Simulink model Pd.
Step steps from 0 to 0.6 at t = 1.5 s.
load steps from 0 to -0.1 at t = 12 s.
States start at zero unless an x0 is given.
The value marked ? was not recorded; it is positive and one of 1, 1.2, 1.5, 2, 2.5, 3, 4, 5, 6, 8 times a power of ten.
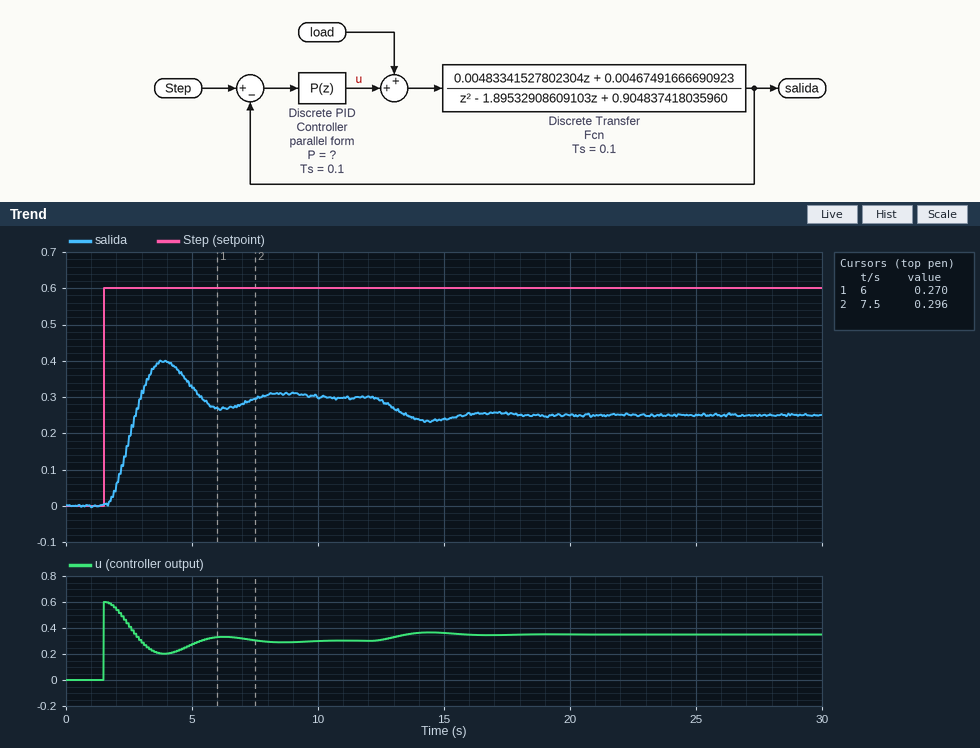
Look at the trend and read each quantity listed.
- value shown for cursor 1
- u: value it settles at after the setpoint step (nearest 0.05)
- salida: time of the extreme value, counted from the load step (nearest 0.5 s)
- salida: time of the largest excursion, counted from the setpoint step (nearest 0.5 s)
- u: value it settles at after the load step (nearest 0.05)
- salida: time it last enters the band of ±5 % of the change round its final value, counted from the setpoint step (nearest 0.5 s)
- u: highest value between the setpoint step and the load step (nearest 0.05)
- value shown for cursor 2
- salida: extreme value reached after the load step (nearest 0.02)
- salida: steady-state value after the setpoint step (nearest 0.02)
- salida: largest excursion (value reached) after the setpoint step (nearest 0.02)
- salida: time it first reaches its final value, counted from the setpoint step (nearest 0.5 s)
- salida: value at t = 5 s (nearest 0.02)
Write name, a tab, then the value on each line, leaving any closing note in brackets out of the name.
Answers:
value shown for cursor 1	0.270
u: value it settles at after the setpoint step	0.30
salida: time of the extreme value, counted from the load step	2.5 s
salida: time of the largest excursion, counted from the setpoint step	2.5 s
u: value it settles at after the load step	0.35
salida: time it last enters the band of ±5 % of the change round its final value, counted from the setpoint step	5.5 s
u: highest value between the setpoint step and the load step	0.60
value shown for cursor 2	0.296
salida: extreme value reached after the load step	0.24
salida: steady-state value after the setpoint step	0.30
salida: largest excursion (value reached) after the setpoint step	0.40
salida: time it first reaches its final value, counted from the setpoint step	1.5 s
salida: value at t = 5 s	0.32
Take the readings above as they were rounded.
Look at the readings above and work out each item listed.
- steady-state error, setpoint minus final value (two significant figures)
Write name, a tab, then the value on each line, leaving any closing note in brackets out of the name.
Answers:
steady-state error, setpoint minus final value	0.30
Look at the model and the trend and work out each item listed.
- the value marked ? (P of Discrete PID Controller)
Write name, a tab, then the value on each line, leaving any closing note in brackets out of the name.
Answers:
the value marked ?	1
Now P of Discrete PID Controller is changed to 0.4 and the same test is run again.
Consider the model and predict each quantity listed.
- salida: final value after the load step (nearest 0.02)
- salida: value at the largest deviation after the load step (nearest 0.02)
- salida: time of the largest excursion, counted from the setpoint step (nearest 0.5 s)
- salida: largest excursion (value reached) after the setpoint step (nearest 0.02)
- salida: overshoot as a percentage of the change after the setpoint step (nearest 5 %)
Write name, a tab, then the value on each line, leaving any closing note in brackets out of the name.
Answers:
salida: final value after the load step	0.10
salida: value at the largest deviation after the load step	0.08
salida: time of the largest excursion, counted from the setpoint step	3.0 s
salida: largest excursion (value reached) after the setpoint step	0.22
salida: overshoot as a percentage of the change after the setpoint step	25 %
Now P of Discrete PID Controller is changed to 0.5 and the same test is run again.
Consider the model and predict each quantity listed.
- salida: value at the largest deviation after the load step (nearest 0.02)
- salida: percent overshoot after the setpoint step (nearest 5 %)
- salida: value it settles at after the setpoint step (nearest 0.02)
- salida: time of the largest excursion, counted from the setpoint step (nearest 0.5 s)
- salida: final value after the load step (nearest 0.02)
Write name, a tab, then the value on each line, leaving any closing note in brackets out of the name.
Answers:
salida: value at the largest deviation after the load step	0.12
salida: percent overshoot after the setpoint step	25 %
salida: value it settles at after the setpoint step	0.20
salida: time of the largest excursion, counted from the setpoint step	3.0 s
salida: final value after the load step	0.14
